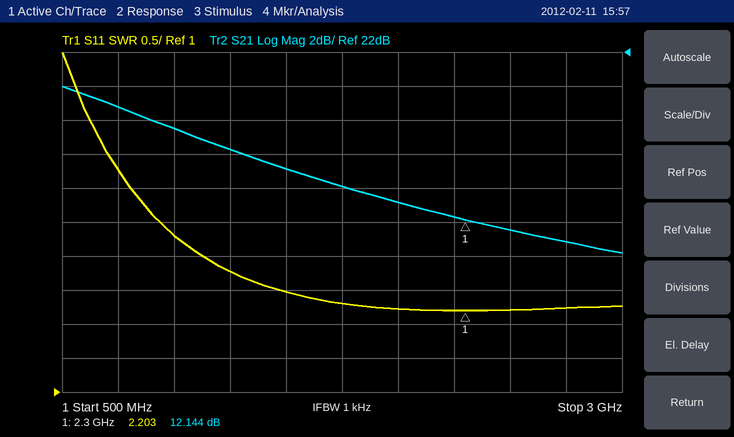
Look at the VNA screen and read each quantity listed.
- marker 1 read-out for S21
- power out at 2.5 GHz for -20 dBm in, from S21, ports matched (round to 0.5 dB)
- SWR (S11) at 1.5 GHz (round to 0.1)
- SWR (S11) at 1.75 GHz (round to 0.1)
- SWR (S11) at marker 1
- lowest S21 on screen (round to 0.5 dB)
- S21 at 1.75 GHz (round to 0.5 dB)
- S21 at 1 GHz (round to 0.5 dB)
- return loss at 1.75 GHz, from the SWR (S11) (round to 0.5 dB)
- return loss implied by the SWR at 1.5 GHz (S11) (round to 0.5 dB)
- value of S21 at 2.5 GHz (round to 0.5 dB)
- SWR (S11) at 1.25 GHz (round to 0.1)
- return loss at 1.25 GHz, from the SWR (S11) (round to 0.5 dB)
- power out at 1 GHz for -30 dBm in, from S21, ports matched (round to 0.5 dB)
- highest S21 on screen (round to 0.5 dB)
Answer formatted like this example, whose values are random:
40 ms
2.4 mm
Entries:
12.144 dB
-8.5 dBm
2.5
2.3
2.203
10.0 dB
14.0 dB
17.5 dB
8.0 dB
7.5 dB
11.5 dB
2.8
6.5 dB
-12.5 dBm
20.0 dB
